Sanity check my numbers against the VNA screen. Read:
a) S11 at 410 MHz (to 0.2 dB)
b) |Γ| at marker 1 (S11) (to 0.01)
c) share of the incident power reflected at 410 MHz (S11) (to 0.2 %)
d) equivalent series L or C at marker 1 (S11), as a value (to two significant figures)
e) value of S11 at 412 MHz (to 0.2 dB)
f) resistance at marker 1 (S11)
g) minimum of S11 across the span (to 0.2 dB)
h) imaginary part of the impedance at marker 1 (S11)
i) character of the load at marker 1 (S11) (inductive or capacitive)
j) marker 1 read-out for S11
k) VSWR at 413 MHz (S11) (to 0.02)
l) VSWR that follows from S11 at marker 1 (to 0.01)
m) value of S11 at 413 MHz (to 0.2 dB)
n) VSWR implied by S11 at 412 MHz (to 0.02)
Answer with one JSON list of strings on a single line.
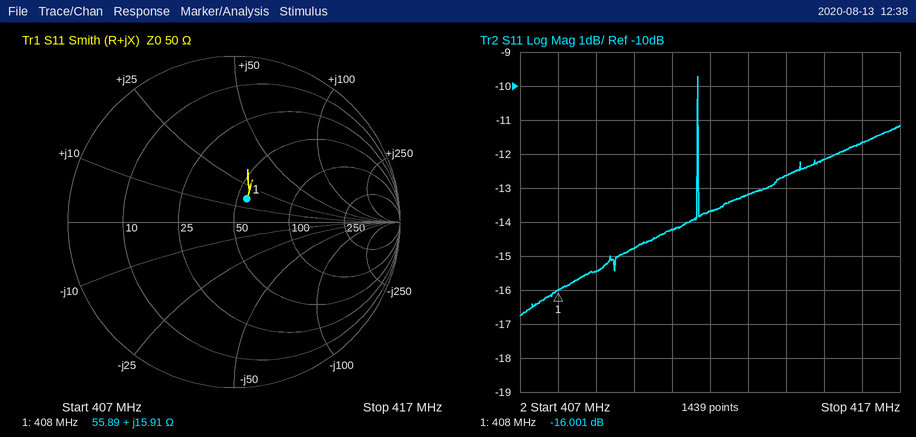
["-14.8 dB", "0.16", "3.4 %", "6.2 nH", "-13.6 dB", "55.89 Ω", "-16.8 dB", "+15.91 Ω", "inductive", "-16.001 dB", "1.56", "1.38", "-13.2 dB", "1.52"]
